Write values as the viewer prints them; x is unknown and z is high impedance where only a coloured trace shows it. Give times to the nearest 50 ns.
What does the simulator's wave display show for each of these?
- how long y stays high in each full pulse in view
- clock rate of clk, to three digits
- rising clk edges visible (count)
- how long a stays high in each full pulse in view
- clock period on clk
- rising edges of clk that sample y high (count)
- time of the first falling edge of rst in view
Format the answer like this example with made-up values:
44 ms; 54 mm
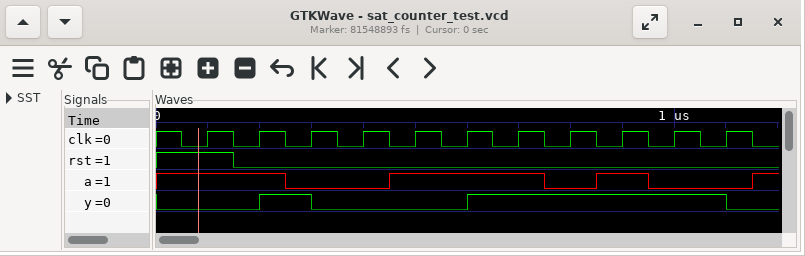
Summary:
100 ns, 500 ns; 10.0 MHz; 11; 300 ns, 100 ns; 100 ns; 6; 150 ns
